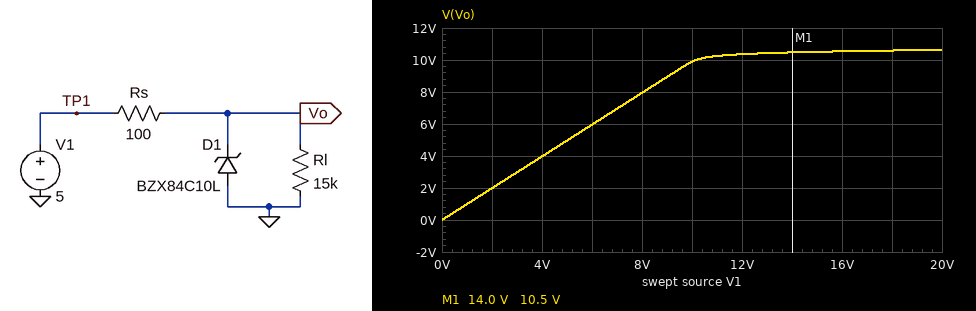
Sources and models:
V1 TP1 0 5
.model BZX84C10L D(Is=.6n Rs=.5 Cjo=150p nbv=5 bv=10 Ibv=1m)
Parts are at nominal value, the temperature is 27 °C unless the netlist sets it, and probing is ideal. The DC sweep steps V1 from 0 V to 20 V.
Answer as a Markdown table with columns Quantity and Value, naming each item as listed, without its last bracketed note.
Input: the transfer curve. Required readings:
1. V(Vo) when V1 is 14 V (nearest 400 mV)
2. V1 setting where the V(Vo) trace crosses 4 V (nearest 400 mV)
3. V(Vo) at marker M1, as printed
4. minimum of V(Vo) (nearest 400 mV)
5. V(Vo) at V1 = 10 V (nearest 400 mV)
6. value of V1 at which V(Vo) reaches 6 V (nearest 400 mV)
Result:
| Quantity | Value |
|---|---|
| V(Vo) when V1 is 14 V | 10.4 V |
| V1 setting where the V(Vo) trace crosses 4 V | 4.0 V |
| V(Vo) at marker M1, as printed | 10.5 V |
| minimum of V(Vo) | 0 V |
| V(Vo) at V1 = 10 V | 10.0 V |
| value of V1 at which V(Vo) reaches 6 V | 6.0 V |
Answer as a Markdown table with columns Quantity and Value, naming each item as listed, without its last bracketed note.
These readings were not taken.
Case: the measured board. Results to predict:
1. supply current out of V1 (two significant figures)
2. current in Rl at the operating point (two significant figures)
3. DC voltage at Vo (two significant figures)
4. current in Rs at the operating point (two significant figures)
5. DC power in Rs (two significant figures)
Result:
| Quantity | Value |
|---|---|
| supply current out of V1 | 330 µA |
| current in Rl at the operating point | 330 µA |
| DC voltage at Vo | 5.0 V |
| current in Rs at the operating point | 330 µA |
| DC power in Rs | 11 µW |
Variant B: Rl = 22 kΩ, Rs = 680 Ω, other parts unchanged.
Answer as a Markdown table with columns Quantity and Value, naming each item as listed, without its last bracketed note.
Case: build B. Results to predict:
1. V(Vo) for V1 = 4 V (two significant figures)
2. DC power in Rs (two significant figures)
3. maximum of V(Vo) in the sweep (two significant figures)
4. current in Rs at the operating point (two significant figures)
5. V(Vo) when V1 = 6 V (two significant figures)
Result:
| Quantity | Value |
|---|---|
| V(Vo) for V1 = 4 V | 3.9 V |
| DC power in Rs | 33 µW |
| maximum of V(Vo) in the sweep | 10 V |
| current in Rs at the operating point | 220 µA |
| V(Vo) when V1 = 6 V | 5.8 V |
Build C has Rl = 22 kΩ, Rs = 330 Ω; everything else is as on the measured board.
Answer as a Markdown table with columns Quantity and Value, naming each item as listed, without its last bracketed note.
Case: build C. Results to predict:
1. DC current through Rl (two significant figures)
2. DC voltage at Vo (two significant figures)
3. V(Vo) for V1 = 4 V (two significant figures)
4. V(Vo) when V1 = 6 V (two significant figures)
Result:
| Quantity | Value |
|---|---|
| DC current through Rl | 220 µA |
| DC voltage at Vo | 4.9 V |
| V(Vo) for V1 = 4 V | 3.9 V |
| V(Vo) when V1 = 6 V | 5.9 V |
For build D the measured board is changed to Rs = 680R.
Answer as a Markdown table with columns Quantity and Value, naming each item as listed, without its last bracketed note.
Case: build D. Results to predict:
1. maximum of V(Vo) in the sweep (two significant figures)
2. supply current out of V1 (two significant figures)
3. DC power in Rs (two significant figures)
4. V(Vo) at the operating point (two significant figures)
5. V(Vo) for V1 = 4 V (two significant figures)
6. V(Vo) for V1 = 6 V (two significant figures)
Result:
| Quantity | Value |
|---|---|
| maximum of V(Vo) in the sweep | 10 V |
| supply current out of V1 | 320 µA |
| DC power in Rs | 69 µW |
| V(Vo) at the operating point | 4.8 V |
| V(Vo) for V1 = 4 V | 3.8 V |
| V(Vo) for V1 = 6 V | 5.7 V |
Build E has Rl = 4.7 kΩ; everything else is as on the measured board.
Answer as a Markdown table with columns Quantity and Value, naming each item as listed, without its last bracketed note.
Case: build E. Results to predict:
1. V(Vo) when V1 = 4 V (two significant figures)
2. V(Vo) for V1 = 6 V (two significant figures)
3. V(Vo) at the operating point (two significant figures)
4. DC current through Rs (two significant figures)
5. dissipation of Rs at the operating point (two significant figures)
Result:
| Quantity | Value |
|---|---|
| V(Vo) when V1 = 4 V | 3.9 V |
| V(Vo) for V1 = 6 V | 5.9 V |
| V(Vo) at the operating point | 4.9 V |
| DC current through Rs | 1.0 mA |
| dissipation of Rs at the operating point | 110 µW |
